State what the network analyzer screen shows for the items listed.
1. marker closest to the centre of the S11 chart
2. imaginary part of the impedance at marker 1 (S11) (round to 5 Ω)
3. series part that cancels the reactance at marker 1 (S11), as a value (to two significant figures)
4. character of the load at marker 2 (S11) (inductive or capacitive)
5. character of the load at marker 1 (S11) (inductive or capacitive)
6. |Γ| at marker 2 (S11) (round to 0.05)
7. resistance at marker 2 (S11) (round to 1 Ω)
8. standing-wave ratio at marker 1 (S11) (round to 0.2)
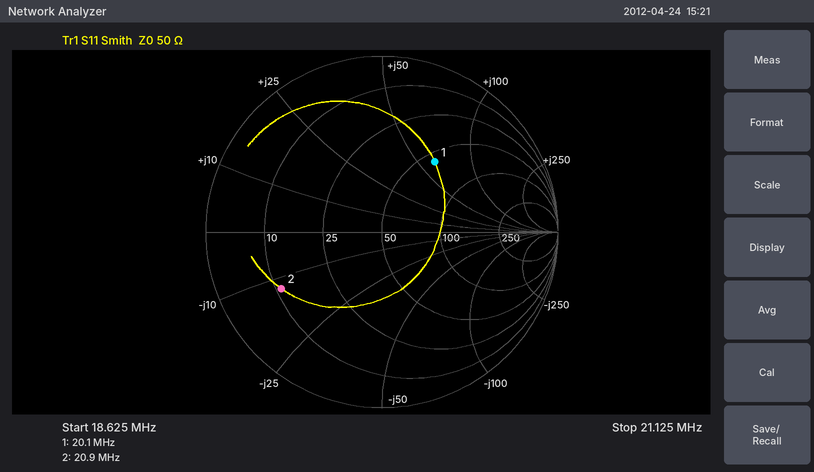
marker 1
+60 Ω
130 pF
capacitive
inductive
0.65
11 Ω
3.0
